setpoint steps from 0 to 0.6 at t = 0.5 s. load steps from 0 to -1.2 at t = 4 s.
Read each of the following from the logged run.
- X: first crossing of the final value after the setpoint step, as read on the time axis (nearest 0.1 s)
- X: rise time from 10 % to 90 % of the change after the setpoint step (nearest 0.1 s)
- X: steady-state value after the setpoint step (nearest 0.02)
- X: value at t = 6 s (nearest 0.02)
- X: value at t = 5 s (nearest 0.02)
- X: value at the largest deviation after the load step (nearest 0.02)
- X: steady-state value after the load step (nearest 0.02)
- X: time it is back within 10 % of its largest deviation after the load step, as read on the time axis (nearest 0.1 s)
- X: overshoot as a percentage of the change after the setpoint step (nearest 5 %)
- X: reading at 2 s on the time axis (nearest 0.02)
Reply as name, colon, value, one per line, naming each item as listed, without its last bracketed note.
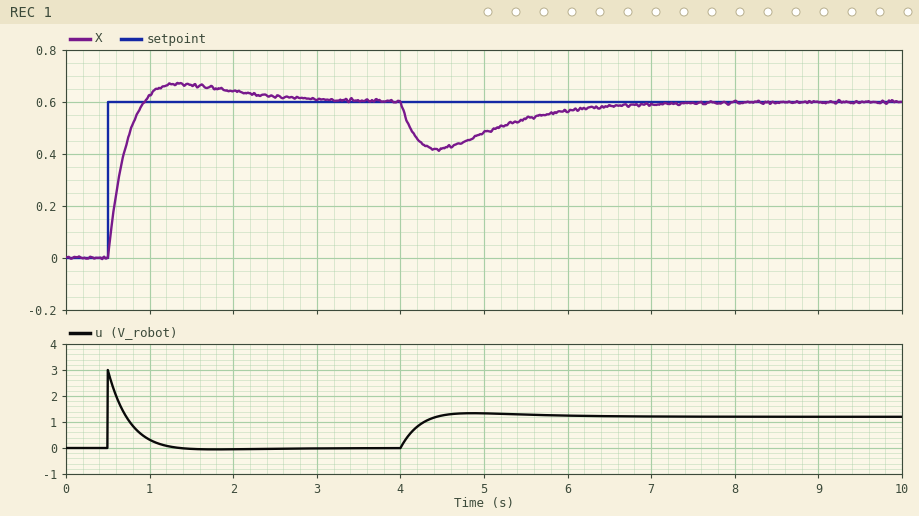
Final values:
X: first crossing of the final value after the setpoint step, as read on the time axis: 0.9 s
X: rise time from 10 % to 90 % of the change after the setpoint step: 0.3 s
X: steady-state value after the setpoint step: 0.60
X: value at t = 6 s: 0.56
X: value at t = 5 s: 0.48
X: value at the largest deviation after the load step: 0.42
X: steady-state value after the load step: 0.60
X: time it is back within 10 % of its largest deviation after the load step, as read on the time axis: 6.4 s
X: overshoot as a percentage of the change after the setpoint step: 10 %
X: reading at 2 s on the time axis: 0.64
